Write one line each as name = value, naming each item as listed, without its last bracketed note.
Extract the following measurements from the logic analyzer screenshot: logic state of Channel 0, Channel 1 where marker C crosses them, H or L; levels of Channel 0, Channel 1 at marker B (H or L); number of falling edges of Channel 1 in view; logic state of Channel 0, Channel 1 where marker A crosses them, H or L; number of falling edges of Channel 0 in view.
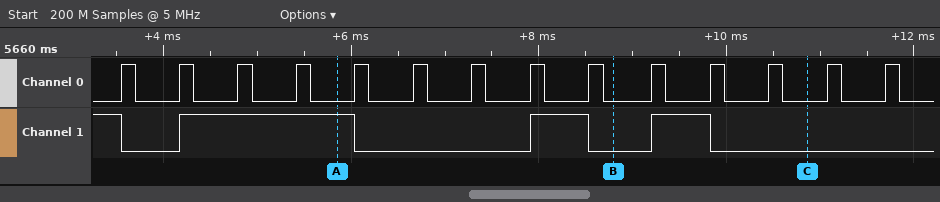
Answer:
logic state of Channel 0, Channel 1 where marker C crosses them, H or L = Channel 0=L, Channel 1=L
levels of Channel 0, Channel 1 at marker B = Channel 0=L, Channel 1=L
number of falling edges of Channel 1 in view = 4
logic state of Channel 0, Channel 1 where marker A crosses them, H or L = Channel 0=L, Channel 1=H
number of falling edges of Channel 0 in view = 14
